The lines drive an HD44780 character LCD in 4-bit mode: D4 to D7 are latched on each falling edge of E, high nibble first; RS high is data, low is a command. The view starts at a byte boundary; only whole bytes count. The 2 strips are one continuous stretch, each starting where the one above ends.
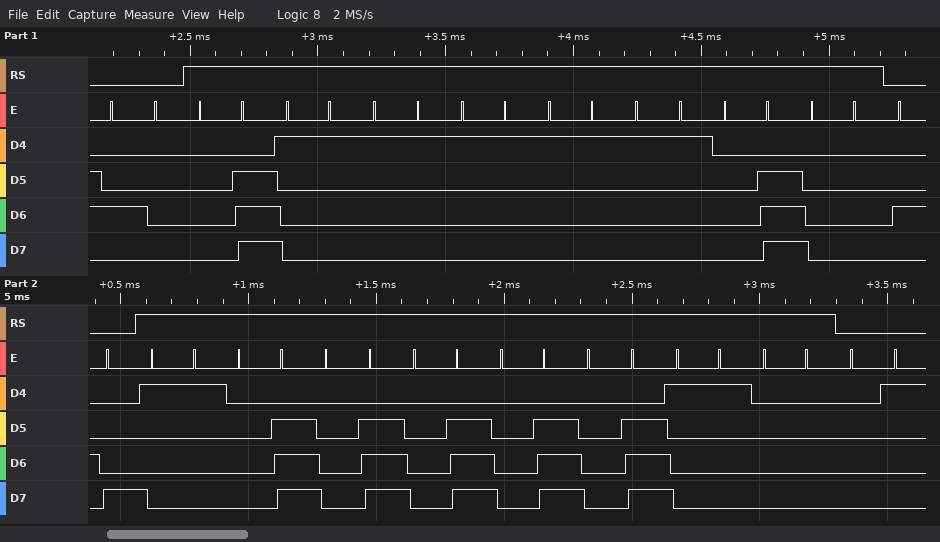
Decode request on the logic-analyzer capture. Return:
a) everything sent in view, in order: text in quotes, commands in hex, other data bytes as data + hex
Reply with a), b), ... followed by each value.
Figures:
a) 0x40 data 0E 11 11 11 11 11 0E 00 0x48 data 11 0E 0E 0E 0E 0E 11 00 0x01
